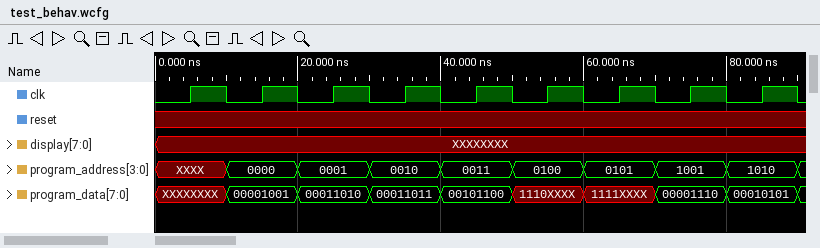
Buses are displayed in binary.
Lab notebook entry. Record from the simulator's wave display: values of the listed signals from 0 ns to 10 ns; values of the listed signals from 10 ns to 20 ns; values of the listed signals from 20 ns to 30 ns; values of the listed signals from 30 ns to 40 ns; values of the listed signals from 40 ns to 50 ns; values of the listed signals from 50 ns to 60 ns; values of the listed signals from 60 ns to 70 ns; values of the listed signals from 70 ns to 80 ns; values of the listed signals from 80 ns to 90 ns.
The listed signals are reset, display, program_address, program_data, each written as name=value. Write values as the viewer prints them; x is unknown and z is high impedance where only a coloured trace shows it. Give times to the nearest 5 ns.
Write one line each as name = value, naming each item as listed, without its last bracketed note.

values of the listed signals from 0 ns to 10 ns = reset=x, display=XXXXXXXX, program_address=XXXX, program_data=XXXXXXXX
values of the listed signals from 10 ns to 20 ns = reset=x, display=XXXXXXXX, program_address=0000, program_data=00001001
values of the listed signals from 20 ns to 30 ns = reset=x, display=XXXXXXXX, program_address=0001, program_data=00011010
values of the listed signals from 30 ns to 40 ns = reset=x, display=XXXXXXXX, program_address=0010, program_data=00011011
values of the listed signals from 40 ns to 50 ns = reset=x, display=XXXXXXXX, program_address=0011, program_data=00101100
values of the listed signals from 50 ns to 60 ns = reset=x, display=XXXXXXXX, program_address=0100, program_data=1110XXXX
values of the listed signals from 60 ns to 70 ns = reset=x, display=XXXXXXXX, program_address=0101, program_data=1111XXXX
values of the listed signals from 70 ns to 80 ns = reset=x, display=XXXXXXXX, program_address=1001, program_data=00001110
values of the listed signals from 80 ns to 90 ns = reset=x, display=XXXXXXXX, program_address=1010, program_data=00010101
